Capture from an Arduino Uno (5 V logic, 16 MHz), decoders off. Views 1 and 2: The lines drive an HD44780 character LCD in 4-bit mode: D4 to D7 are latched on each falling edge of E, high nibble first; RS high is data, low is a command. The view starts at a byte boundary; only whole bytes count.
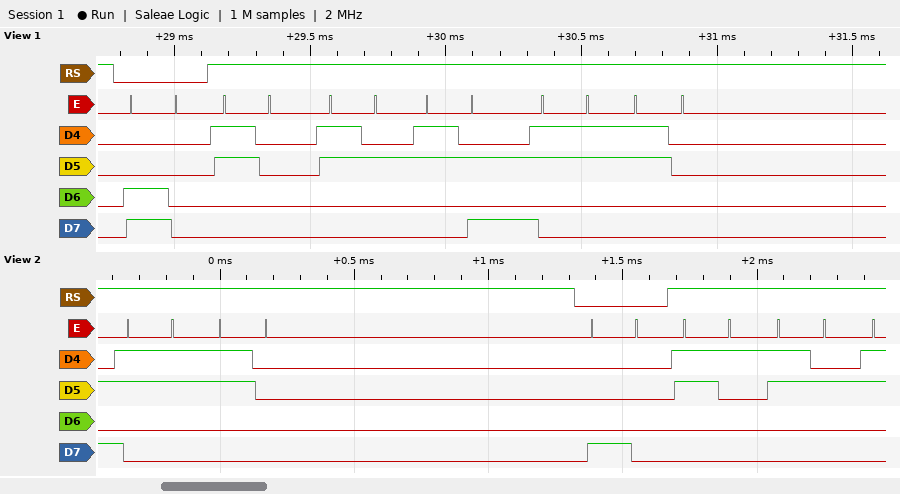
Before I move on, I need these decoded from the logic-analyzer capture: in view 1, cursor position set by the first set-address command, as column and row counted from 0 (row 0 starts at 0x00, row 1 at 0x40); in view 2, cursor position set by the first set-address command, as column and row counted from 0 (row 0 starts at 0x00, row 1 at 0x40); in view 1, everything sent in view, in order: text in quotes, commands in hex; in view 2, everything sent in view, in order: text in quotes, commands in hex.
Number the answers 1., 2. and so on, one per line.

1. column 0, row 1
2. column 0, row 0
3. 0xC0 "02:30"
4. "30" 0x80 "12"
